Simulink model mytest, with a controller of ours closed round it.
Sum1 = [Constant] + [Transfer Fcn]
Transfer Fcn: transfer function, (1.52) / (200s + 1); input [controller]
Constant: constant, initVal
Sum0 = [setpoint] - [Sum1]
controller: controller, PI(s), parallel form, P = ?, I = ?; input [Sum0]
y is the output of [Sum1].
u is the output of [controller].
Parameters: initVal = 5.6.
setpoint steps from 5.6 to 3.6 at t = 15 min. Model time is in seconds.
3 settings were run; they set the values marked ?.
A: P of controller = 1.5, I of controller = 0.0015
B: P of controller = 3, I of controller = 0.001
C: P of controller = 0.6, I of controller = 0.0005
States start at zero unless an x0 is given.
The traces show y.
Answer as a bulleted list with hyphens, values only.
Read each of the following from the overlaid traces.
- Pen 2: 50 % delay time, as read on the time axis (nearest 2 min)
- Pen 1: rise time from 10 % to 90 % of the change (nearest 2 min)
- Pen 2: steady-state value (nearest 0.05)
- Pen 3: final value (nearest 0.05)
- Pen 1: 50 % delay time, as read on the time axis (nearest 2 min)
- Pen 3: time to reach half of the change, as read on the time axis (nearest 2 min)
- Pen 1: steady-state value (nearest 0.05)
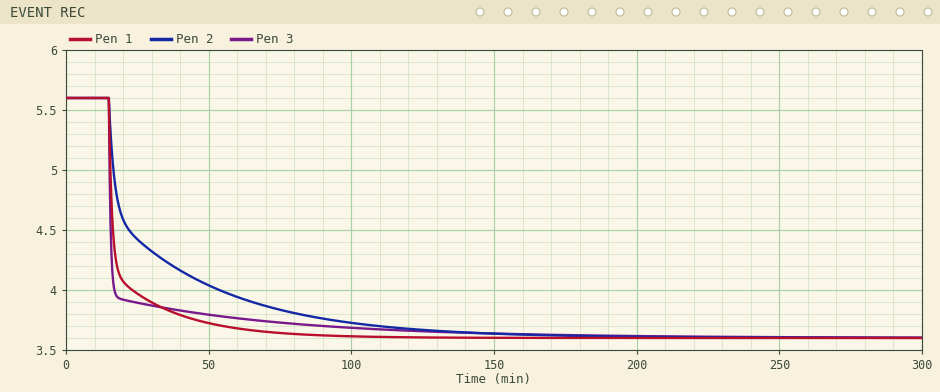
- 20 min
- 24 min
- 3.60
- 3.60
- 16 min
- 16 min
- 3.60
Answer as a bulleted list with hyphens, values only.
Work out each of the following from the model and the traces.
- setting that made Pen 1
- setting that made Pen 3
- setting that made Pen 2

- A
- B
- C
